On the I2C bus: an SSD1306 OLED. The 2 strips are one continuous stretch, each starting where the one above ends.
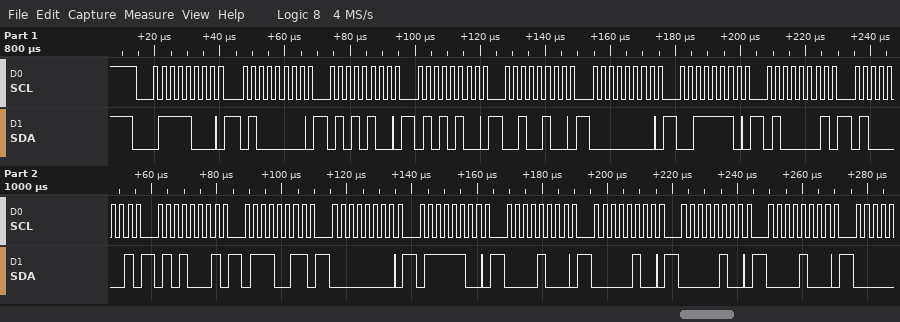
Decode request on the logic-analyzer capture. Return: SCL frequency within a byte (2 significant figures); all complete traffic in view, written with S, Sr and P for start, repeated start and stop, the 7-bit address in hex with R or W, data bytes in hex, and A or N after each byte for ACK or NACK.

400 kHz
S 3CW A 40 A 54 A 54 A 24 A 00 A 3E A 41 A 41 A 51 A 73 A 00 A 7C A 08 A 04 A 04 A 08 A
